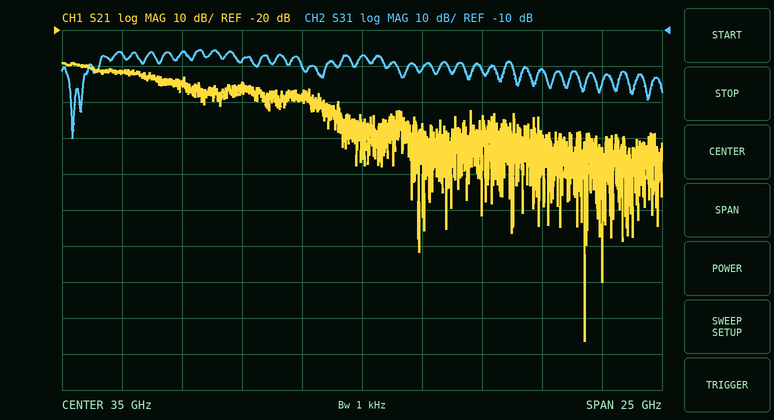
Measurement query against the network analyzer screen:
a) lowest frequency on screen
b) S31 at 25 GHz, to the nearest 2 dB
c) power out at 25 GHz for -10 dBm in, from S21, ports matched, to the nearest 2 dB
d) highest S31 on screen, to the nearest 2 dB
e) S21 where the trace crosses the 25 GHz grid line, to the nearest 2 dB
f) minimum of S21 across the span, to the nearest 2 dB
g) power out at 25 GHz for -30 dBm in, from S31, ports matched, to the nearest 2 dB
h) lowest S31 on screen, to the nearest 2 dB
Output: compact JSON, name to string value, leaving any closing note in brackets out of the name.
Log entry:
{"lowest frequency on screen": "22.5 GHz", "S31 at 25 GHz, to the nearest 2 dB": "-16 dB", "power out at 25 GHz for -10 dBm in, from S21, ports matched, to the nearest 2 dB": "-42 dBm", "highest S31 on screen, to the nearest 2 dB": "-16 dB", "S21 where the trace crosses the 25 GHz grid line, to the nearest 2 dB": "-32 dB", "minimum of S21 across the span, to the nearest 2 dB": "-106 dB", "power out at 25 GHz for -30 dBm in, from S31, ports matched, to the nearest 2 dB": "-46 dBm", "lowest S31 on screen, to the nearest 2 dB": "-40 dB"}
